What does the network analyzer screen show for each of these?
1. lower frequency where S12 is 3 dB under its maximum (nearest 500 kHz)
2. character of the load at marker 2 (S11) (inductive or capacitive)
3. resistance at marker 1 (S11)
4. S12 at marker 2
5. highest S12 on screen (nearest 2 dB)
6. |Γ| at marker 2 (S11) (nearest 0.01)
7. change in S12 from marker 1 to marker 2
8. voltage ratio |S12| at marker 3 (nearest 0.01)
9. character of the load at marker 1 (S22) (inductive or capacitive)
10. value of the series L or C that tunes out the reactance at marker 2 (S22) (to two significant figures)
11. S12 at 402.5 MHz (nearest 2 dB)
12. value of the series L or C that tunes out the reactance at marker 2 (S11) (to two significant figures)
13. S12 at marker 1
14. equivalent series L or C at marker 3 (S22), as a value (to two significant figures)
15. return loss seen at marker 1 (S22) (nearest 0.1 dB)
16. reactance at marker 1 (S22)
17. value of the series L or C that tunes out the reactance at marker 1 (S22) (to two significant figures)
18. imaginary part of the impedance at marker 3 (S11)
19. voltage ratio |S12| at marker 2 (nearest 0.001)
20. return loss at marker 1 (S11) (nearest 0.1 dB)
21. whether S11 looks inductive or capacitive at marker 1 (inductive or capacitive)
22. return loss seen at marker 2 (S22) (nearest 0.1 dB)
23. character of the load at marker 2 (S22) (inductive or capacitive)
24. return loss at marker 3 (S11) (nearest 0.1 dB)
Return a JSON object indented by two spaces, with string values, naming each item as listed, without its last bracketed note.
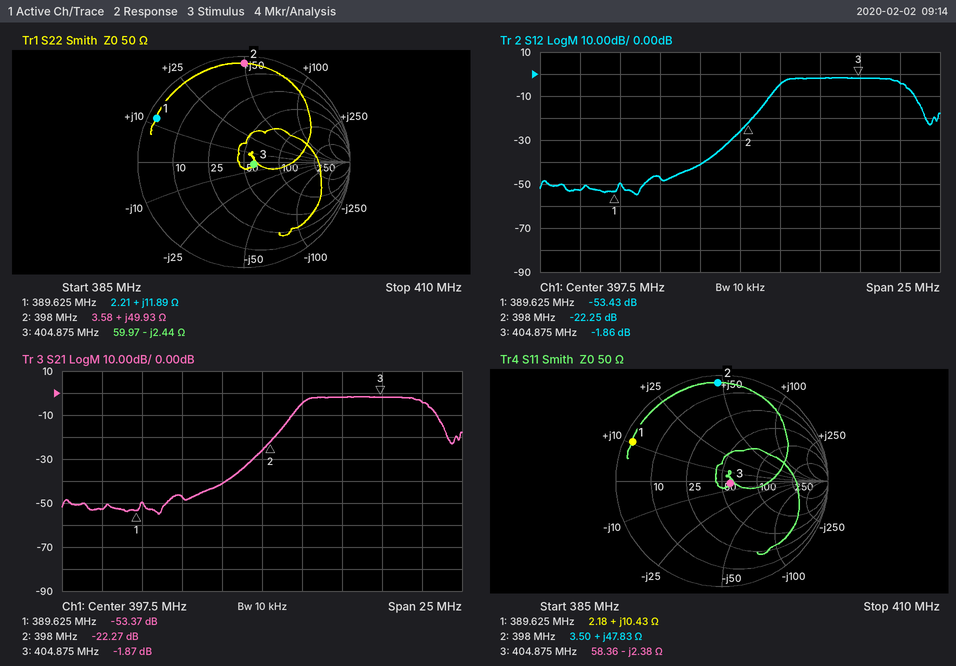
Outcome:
{
  "lower frequency where S12 is 3 dB under its maximum": "400.0 MHz",
  "character of the load at marker 2 (S11)": "inductive",
  "resistance at marker 1": "2.18 Ω",
  "S12 at marker 2": "-22.25 dB",
  "highest S12 on screen": "-2 dB",
  "|Γ| at marker 2 (S11)": "0.93",
  "change in S12 from marker 1 to marker 2": "31.18 dB",
  "voltage ratio |S12| at marker 3": "0.81",
  "character of the load at marker 1 (S22)": "inductive",
  "value of the series L or C that tunes out the reactance at marker 2 (S22)": "8.0 pF",
  "S12 at 402.5 MHz": "-2 dB",
  "value of the series L or C that tunes out the reactance at marker 2 (S11)": "8.4 pF",
  "S12 at marker 1": "-53.43 dB",
  "equivalent series L or C at marker 3 (S22), as a value": "160 pF",
  "return loss seen at marker 1 (S22)": "0.7 dB",
  "reactance at marker 1": "+11.89 Ω",
  "value of the series L or C that tunes out the reactance at marker 1 (S22)": "34 pF",
  "imaginary part of the impedance at marker 3": "-2.38 Ω",
  "voltage ratio |S12| at marker 2": "0.077",
  "return loss at marker 1 (S11)": "0.7 dB",
  "whether S11 looks inductive or capacitive at marker 1": "inductive",
  "return loss seen at marker 2 (S22)": "0.6 dB",
  "character of the load at marker 2 (S22)": "inductive",
  "return loss at marker 3 (S11)": "21.9 dB"
}
